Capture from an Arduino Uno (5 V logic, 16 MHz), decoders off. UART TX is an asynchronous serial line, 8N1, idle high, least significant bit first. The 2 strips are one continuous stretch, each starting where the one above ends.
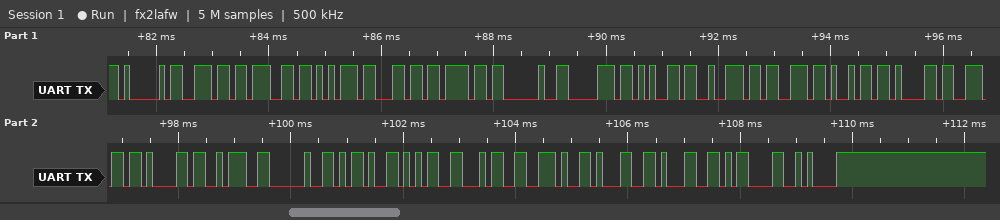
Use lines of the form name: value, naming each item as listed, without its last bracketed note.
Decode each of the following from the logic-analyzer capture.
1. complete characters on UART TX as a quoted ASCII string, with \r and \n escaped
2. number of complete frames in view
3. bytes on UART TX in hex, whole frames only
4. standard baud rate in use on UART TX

complete characters on UART TX as a quoted ASCII string, with \r and \n escaped: "Angulo persiana: -54.11\r\n"
number of complete frames in view: 25
bytes on UART TX in hex, whole frames only: 0x41 0x6E 0x67 0x75 0x6C 0x6F 0x20 0x70 0x65 0x72 0x73 0x69 0x61 0x6E 0x61 0x3A 0x20 0x2D 0x35 0x34 0x2E 0x31 0x31 0x0D 0x0A
standard baud rate in use on UART TX: 9600 baud
